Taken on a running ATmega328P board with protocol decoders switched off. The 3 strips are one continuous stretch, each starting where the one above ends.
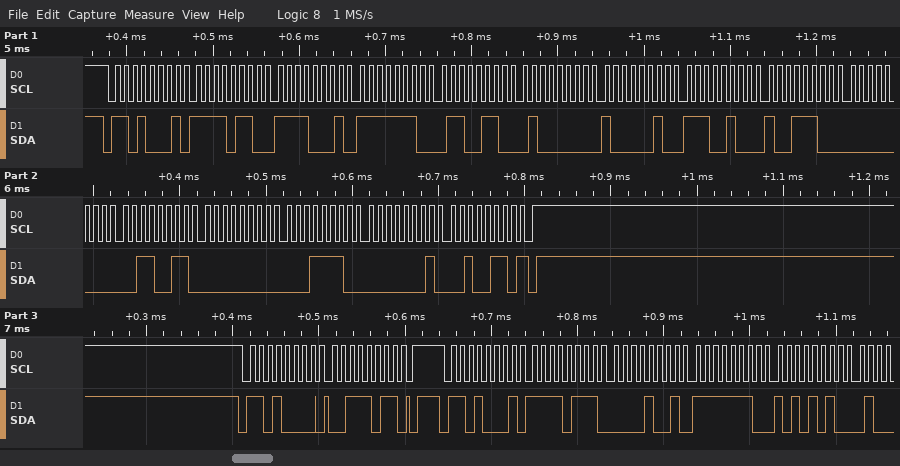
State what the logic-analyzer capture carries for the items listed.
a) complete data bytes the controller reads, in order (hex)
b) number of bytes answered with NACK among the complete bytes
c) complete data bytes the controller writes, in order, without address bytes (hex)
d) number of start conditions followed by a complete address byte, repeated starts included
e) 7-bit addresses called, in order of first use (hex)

F6 F1 FE 66 40 82 E4 9C 00 33 00 1E 01 26 F7 09 FE AA
1
3B
3
0x68
